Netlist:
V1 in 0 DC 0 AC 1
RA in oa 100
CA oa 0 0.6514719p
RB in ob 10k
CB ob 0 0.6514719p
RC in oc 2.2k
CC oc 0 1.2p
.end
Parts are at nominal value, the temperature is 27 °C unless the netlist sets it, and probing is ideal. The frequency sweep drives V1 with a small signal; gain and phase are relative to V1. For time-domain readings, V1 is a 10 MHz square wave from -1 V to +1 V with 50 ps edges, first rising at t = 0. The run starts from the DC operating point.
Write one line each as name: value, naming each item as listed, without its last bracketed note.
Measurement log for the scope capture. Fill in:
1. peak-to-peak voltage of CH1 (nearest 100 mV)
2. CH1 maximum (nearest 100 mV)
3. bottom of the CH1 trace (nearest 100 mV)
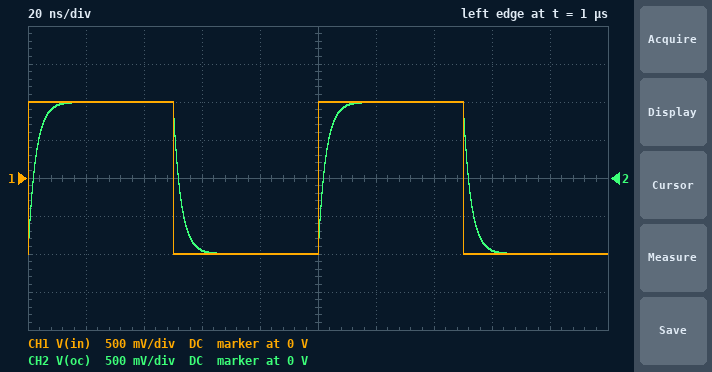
peak-to-peak voltage of CH1: 2.0 V
CH1 maximum: 1.0 V
bottom of the CH1 trace: -1.0 V
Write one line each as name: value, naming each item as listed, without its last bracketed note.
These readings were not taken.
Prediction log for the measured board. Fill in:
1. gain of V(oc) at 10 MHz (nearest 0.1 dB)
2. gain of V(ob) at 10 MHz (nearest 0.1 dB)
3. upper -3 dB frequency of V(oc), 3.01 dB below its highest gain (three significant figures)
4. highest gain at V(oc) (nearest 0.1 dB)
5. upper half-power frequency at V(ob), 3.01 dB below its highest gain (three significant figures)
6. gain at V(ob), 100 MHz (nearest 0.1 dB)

gain of V(oc) at 10 MHz: -0.1 dB
gain of V(ob) at 10 MHz: -0.7 dB
upper -3 dB frequency of V(oc), 3.01 dB below its highest gain: 60.3 MHz
highest gain at V(oc): 0 dB
upper half-power frequency at V(ob), 3.01 dB below its highest gain: 24.4 MHz
gain at V(ob), 100 MHz: -12.5 dB
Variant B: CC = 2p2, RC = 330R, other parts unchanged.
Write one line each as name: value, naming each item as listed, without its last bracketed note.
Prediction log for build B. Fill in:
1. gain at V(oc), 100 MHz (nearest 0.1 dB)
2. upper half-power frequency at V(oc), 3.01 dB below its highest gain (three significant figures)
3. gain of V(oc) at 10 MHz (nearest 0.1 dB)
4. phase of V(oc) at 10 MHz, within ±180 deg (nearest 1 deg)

gain at V(oc), 100 MHz: -0.8 dB
upper half-power frequency at V(oc), 3.01 dB below its highest gain: 219 MHz
gain of V(oc) at 10 MHz: 0 dB
phase of V(oc) at 10 MHz, within ±180 deg: -3 deg
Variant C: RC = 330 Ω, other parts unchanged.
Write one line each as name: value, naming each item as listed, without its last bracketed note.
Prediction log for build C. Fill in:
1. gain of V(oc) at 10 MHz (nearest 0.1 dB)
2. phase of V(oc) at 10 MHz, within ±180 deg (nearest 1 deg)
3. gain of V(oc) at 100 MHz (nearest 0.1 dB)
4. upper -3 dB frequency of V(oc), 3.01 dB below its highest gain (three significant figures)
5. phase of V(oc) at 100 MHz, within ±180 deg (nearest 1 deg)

gain of V(oc) at 10 MHz: 0 dB
phase of V(oc) at 10 MHz, within ±180 deg: -1 deg
gain of V(oc) at 100 MHz: -0.3 dB
upper -3 dB frequency of V(oc), 3.01 dB below its highest gain: 402 MHz
phase of V(oc) at 100 MHz, within ±180 deg: -14 deg
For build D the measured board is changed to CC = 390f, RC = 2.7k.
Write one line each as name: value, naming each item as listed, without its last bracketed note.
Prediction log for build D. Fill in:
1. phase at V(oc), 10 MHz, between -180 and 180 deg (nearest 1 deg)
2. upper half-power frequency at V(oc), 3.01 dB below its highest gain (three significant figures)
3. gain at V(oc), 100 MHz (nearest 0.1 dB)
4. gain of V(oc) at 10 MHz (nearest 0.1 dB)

phase at V(oc), 10 MHz, between -180 and 180 deg: -4 deg
upper half-power frequency at V(oc), 3.01 dB below its highest gain: 151 MHz
gain at V(oc), 100 MHz: -1.6 dB
gain of V(oc) at 10 MHz: 0 dB
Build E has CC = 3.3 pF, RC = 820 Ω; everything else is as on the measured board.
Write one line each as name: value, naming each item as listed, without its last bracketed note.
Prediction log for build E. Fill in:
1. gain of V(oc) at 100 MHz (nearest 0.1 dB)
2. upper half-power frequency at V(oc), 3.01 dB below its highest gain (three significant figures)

gain of V(oc) at 100 MHz: -5.9 dB
upper half-power frequency at V(oc), 3.01 dB below its highest gain: 58.8 MHz
